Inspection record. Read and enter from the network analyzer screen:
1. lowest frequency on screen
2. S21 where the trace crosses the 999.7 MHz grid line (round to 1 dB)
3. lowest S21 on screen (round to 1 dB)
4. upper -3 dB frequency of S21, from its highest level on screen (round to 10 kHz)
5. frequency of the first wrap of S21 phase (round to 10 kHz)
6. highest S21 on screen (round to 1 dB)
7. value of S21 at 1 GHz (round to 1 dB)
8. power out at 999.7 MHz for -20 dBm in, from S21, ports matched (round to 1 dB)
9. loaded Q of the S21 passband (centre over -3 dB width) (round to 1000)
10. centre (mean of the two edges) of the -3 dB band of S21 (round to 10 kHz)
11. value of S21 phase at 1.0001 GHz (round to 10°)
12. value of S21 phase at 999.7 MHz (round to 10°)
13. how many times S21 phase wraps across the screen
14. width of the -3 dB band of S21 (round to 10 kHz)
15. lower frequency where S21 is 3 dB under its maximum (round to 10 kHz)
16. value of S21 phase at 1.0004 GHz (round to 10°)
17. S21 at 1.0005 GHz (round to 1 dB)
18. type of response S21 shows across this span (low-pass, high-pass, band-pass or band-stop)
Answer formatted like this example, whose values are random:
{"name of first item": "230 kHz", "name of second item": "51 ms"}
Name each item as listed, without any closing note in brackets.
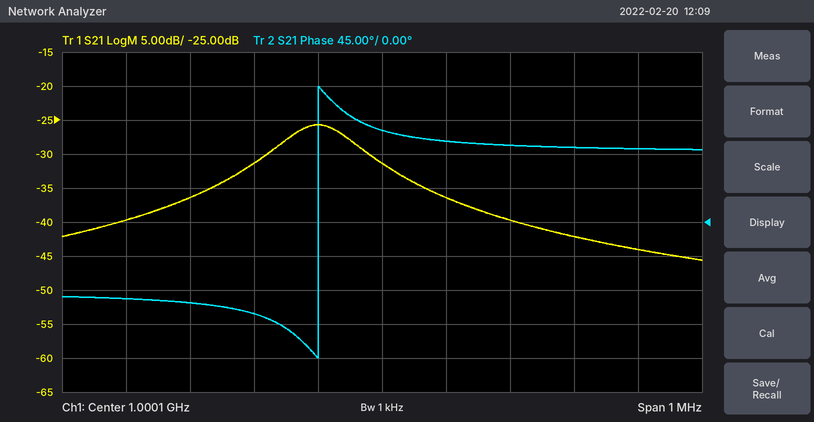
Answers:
{"lowest frequency on screen": "999.6 MHz", "S21 where the trace crosses the 999.7 MHz grid line": "-40 dB", "lowest S21 on screen": "-46 dB", "upper -3 dB frequency of S21, from its highest level on screen": "1.00006 GHz", "frequency of the first wrap of S21 phase": "1.00000 GHz", "highest S21 on screen": "-26 dB", "value of S21 at 1 GHz": "-26 dB", "power out at 999.7 MHz for -20 dBm in, from S21, ports matched": "-60 dBm", "loaded Q of the S21 passband (centre over -3 dB width)": "8000", "centre (mean of the two edges) of the -3 dB band of S21": "1.00000 GHz", "value of S21 phase at 1.0001 GHz": "120°", "value of S21 phase at 999.7 MHz": "-100°", "how many times S21 phase wraps across the screen": "1", "width of the -3 dB band of S21": "120 kHz", "lower frequency where S21 is 3 dB under its maximum": "999.94 MHz", "value of S21 phase at 1.0004 GHz": "100°", "S21 at 1.0005 GHz": "-44 dB", "type of response S21 shows across this span": "band-pass"}
